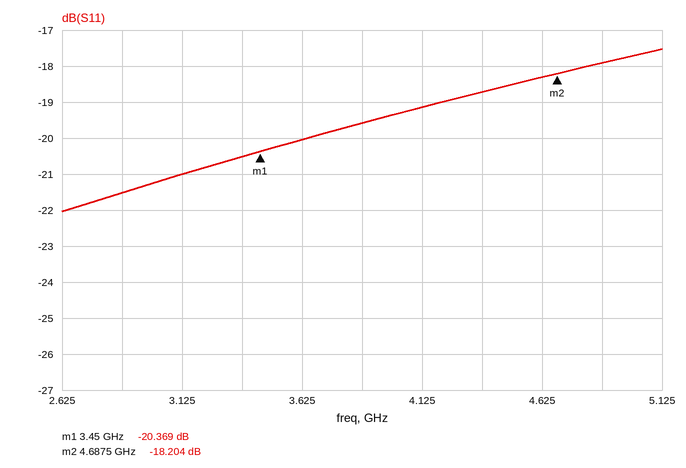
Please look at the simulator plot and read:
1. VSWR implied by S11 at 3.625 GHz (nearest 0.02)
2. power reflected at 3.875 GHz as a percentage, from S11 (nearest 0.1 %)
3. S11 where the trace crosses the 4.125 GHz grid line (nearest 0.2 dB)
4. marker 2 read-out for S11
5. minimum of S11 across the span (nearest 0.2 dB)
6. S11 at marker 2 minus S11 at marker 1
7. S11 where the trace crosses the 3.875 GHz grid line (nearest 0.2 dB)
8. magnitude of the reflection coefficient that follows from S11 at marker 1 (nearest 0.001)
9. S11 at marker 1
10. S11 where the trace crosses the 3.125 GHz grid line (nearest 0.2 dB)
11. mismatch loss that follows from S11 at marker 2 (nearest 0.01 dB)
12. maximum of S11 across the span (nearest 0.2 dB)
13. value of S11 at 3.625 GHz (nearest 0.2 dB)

1.22
1.1 %
-19.2 dB
-18.204 dB
-22.0 dB
2.165 dB
-19.6 dB
0.096
-20.369 dB
-21.0 dB
0.07 dB
-17.6 dB
-20.0 dB
